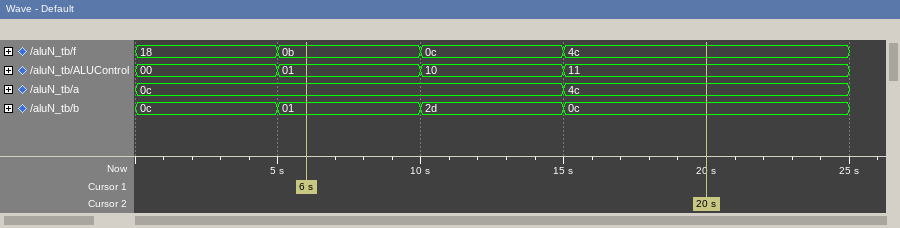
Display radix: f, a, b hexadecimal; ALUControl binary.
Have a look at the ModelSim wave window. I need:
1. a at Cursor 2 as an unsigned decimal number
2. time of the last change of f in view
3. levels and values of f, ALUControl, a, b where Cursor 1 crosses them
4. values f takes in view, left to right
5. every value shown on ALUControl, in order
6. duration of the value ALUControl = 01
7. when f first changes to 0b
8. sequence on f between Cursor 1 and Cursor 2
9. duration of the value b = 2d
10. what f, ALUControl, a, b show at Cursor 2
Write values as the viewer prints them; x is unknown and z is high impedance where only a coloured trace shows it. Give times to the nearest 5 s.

76
15 s
f=0b, ALUControl=01, a=0c, b=01
18, 0b, 0c, 4c
00, 01, 10, 11
5 s
5 s
0b, 0c, 4c
5 s
f=4c, ALUControl=11, a=4c, b=0c
